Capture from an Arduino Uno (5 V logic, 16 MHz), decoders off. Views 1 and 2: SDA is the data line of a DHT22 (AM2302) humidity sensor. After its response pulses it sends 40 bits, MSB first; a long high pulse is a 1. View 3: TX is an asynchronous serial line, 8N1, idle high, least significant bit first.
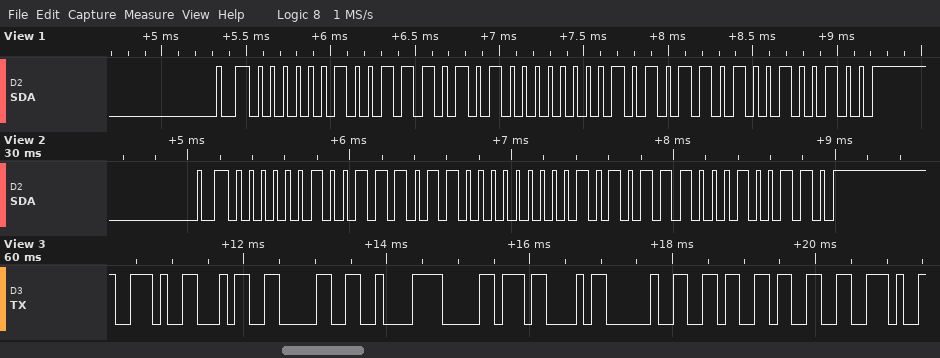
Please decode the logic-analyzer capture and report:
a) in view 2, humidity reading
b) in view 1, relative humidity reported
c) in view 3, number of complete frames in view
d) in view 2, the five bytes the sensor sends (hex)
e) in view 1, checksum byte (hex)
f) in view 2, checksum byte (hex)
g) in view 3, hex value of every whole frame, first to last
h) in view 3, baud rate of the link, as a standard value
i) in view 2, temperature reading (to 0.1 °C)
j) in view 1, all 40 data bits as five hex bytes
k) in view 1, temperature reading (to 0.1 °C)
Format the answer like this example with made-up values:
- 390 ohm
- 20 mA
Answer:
- 63.0 %
- 62.9 %
- 10
- 02 76 00 AE 26
- 0x24
- 0x26
- 0x2E 0x34 0x30 0xC2 0xB0 0x43 0x20 0x36 0x33 0x2E
- 9600 baud
- 17.4 °C
- 02 75 00 AD 24
- 17.3 °C
